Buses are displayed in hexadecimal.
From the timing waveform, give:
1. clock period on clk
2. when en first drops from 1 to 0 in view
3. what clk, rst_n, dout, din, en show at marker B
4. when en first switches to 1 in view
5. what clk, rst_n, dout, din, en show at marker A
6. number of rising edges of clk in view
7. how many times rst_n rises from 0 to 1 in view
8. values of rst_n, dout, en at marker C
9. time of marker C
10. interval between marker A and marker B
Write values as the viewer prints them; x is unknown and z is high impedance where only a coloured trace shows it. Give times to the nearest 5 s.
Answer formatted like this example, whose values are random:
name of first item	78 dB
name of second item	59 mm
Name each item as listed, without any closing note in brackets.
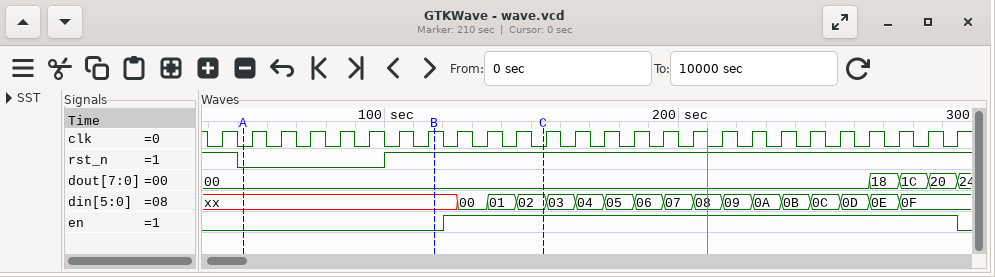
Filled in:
clock period on clk	10 s
when en first drops from 1 to 0 in view	295 s
what clk, rst_n, dout, din, en show at marker B	clk=1, rst_n=1, dout=00, din=xx, en=0
when en first switches to 1 in view	120 s
what clk, rst_n, dout, din, en show at marker A	clk=0, rst_n=0, dout=00, din=xx, en=0
number of rising edges of clk in view	26
how many times rst_n rises from 0 to 1 in view	1
values of rst_n, dout, en at marker C	rst_n=1, dout=00, en=1
time of marker C	155 s
interval between marker A and marker B	65 s
